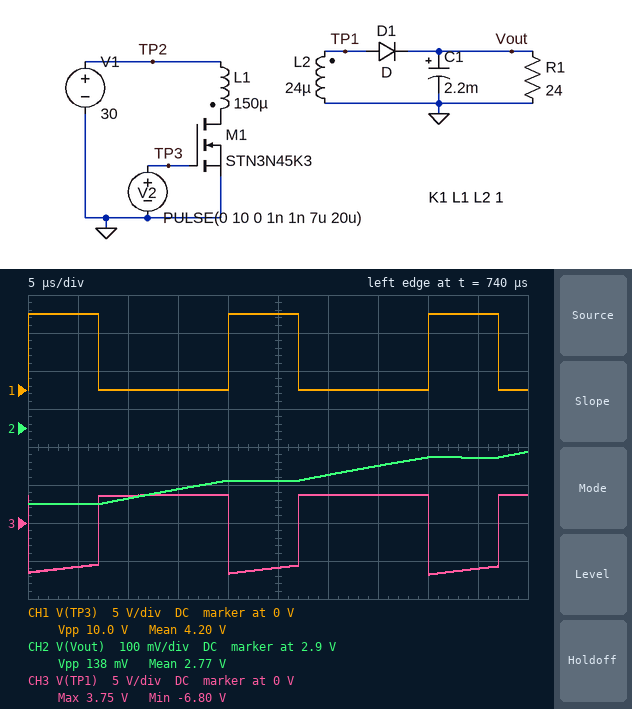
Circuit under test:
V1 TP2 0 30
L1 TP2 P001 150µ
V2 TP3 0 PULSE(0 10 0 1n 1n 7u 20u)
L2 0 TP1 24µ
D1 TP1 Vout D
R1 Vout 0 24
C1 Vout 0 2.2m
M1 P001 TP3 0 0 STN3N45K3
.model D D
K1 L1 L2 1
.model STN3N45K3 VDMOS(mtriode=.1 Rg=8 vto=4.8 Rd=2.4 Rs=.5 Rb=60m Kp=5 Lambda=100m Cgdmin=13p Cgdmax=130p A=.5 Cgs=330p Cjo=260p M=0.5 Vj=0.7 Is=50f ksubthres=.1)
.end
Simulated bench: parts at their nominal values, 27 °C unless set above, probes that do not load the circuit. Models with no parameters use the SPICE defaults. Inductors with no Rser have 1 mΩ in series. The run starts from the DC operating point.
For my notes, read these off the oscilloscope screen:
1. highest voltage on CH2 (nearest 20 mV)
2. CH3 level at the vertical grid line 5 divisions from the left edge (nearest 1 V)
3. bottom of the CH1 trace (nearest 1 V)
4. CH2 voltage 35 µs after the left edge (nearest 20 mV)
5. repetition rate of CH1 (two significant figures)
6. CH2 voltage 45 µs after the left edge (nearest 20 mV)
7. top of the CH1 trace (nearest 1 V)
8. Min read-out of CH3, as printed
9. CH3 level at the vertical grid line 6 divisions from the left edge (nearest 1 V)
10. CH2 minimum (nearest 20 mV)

2.84 V
-6 V
0 V
2.80 V
50 kHz
2.82 V
10 V
-6.80 V
4 V
2.70 V
